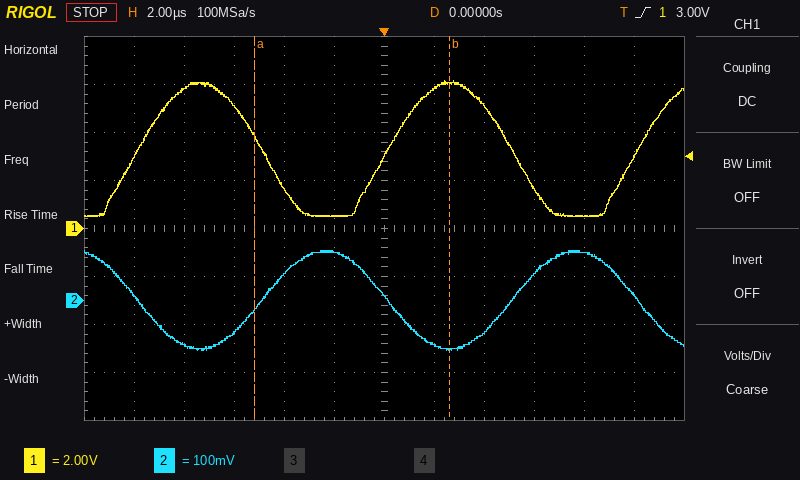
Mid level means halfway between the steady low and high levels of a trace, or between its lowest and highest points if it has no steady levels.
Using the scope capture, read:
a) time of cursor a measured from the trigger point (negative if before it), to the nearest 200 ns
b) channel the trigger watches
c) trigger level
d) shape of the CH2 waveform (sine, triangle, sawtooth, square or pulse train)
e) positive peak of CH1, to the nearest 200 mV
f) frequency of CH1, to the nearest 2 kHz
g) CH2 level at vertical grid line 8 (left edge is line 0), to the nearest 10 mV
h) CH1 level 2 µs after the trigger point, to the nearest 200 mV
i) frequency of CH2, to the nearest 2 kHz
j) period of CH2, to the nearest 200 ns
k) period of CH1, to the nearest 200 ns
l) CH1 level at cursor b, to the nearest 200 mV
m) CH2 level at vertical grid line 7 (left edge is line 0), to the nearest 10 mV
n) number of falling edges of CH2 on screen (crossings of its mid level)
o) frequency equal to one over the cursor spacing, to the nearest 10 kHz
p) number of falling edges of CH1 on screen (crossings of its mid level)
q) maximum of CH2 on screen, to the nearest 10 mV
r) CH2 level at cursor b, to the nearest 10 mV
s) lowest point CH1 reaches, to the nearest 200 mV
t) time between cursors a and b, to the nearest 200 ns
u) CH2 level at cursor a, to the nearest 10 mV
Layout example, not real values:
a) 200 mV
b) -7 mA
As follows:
a) -5.2 µs
b) CH1
c) 3.00 V
d) sine
e) 6.2 V
f) 100 kHz
g) -70 mV
h) 5.8 V
i) 100 kHz
j) 10.0 µs
k) 10.0 µs
l) 6.0 V
m) -90 mV
n) 3
o) 130 kHz
p) 2
q) 100 mV
r) -100 mV
s) 400 mV
t) 7.8 µs
u) -20 mV
